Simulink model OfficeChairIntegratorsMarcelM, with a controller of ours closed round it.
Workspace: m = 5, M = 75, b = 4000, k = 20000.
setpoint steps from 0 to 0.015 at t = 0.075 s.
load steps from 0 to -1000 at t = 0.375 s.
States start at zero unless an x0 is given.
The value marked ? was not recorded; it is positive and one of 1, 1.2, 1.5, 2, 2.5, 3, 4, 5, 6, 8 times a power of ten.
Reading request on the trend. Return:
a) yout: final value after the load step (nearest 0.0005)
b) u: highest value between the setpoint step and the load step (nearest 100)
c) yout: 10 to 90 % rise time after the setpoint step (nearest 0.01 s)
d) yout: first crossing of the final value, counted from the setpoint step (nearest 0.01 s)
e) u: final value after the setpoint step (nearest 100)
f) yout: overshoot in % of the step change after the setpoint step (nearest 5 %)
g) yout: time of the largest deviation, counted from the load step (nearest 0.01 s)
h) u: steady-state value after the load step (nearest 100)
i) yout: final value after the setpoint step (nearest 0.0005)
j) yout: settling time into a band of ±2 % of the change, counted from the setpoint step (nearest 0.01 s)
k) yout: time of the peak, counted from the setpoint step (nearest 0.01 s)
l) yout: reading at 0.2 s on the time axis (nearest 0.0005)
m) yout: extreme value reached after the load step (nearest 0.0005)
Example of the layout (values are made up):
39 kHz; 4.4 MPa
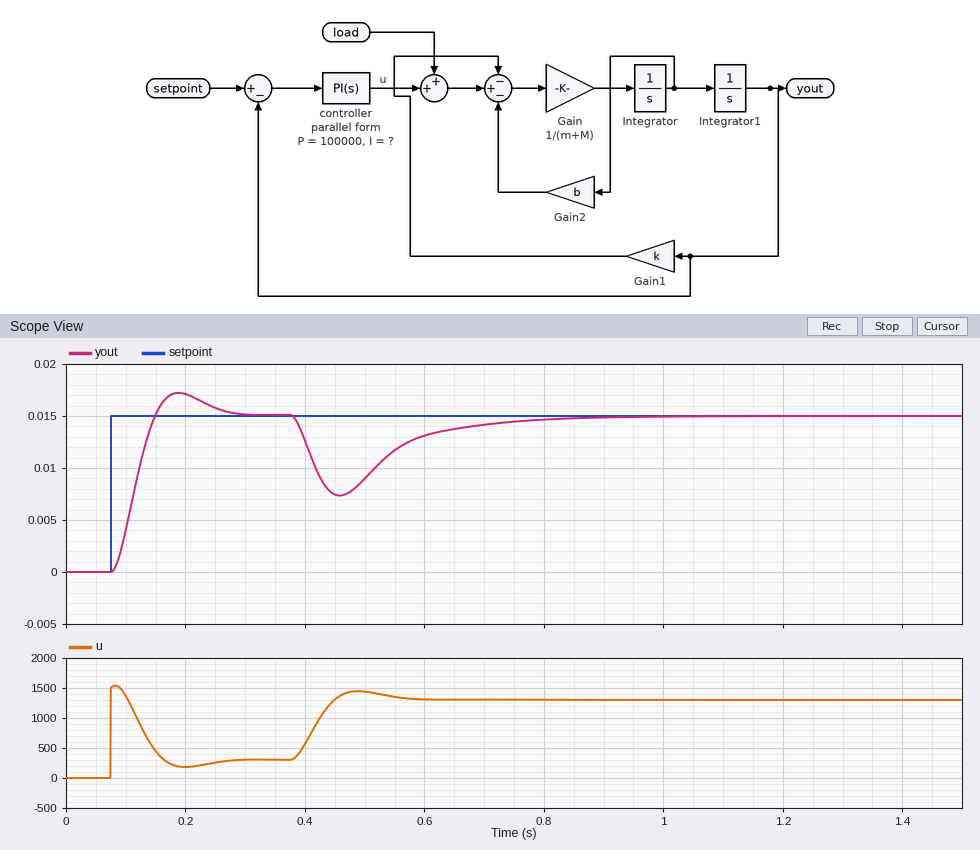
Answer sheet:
0.0150; 1500; 0.05 s; 0.07 s; 300; 15 %; 0.08 s; 1300; 0.0150; 0.20 s; 0.11 s; 0.0170; 0.0075
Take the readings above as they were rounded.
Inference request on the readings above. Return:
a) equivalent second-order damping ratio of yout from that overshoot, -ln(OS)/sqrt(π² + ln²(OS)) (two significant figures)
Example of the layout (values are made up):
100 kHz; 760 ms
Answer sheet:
0.52
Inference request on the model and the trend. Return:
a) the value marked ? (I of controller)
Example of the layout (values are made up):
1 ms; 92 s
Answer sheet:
800000
